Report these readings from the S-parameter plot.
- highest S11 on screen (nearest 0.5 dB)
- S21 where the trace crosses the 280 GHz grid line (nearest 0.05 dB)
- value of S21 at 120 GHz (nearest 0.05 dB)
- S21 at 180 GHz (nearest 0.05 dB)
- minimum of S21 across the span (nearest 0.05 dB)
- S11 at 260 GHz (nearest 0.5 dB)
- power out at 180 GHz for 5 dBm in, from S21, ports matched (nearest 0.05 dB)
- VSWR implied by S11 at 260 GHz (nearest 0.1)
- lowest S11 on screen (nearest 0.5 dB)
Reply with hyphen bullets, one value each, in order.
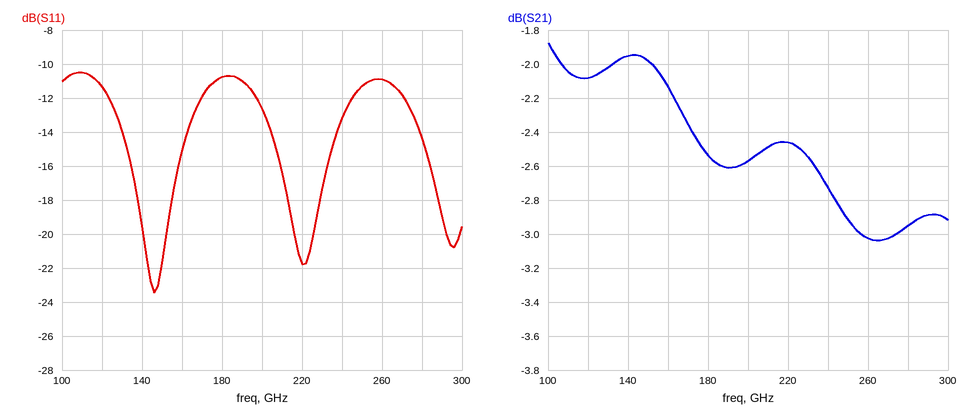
- -10.5 dB
- -2.95 dB
- -2.10 dB
- -2.55 dB
- -3.05 dB
- -11.0 dB
- 2.45 dBm
- 1.8
- -23.5 dB
